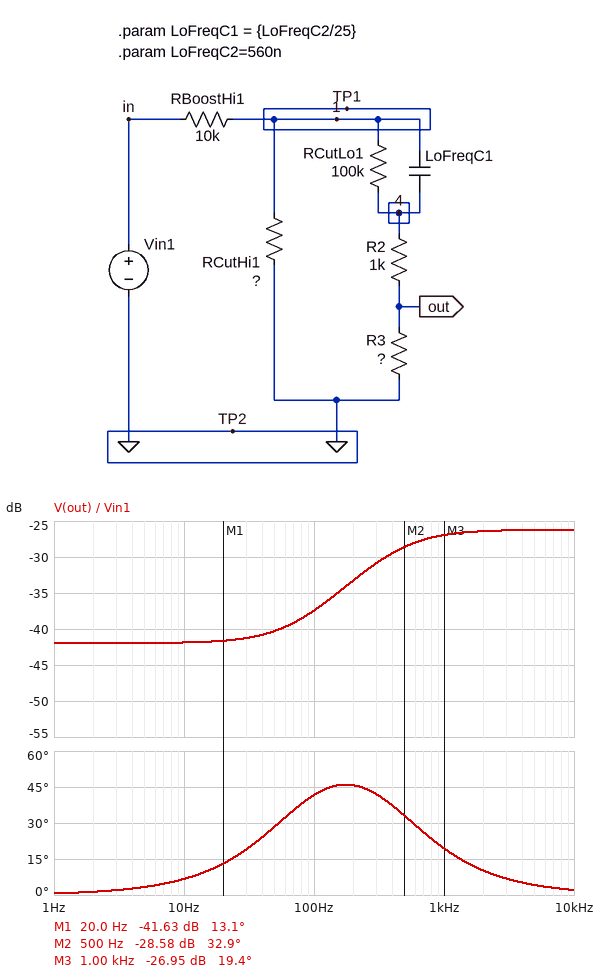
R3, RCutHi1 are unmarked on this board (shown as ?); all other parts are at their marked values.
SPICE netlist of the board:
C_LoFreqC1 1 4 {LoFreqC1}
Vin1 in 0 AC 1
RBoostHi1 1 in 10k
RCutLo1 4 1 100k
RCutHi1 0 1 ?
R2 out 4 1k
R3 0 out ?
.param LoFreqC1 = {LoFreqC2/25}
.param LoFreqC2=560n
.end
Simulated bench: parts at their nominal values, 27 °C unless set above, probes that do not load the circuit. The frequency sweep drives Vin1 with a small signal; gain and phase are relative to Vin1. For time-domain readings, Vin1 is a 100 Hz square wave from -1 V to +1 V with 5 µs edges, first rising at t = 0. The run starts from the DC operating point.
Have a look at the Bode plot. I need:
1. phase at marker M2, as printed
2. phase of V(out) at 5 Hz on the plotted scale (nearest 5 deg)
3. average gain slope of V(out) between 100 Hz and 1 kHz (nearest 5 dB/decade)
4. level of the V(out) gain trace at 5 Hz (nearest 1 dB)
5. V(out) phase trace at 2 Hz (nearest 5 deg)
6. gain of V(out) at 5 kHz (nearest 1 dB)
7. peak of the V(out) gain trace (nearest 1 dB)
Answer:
32.9 deg
5 deg
10 dB/decade
-42 dB
0 deg
-26 dB
-26 dB
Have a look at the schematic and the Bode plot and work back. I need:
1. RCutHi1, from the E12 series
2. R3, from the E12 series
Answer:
560 Ω
18 kΩ
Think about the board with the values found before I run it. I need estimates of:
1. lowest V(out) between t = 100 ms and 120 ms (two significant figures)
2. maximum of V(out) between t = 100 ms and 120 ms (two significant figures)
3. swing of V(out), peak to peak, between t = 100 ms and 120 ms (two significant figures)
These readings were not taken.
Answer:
-89 mV
89 mV
180 mV
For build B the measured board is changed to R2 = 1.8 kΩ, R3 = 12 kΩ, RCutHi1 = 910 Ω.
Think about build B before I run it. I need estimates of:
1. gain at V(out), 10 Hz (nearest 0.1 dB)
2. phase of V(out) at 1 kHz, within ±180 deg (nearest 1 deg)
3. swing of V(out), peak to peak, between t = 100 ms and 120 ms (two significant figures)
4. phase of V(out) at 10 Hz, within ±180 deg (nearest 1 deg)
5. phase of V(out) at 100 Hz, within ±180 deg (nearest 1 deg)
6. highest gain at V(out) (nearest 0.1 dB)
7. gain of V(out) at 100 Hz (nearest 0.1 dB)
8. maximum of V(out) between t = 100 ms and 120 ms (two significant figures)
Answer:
-41.1 dB
25 deg
250 mV
7 deg
44 deg
-23.3 dB
-36.6 dB
130 mV
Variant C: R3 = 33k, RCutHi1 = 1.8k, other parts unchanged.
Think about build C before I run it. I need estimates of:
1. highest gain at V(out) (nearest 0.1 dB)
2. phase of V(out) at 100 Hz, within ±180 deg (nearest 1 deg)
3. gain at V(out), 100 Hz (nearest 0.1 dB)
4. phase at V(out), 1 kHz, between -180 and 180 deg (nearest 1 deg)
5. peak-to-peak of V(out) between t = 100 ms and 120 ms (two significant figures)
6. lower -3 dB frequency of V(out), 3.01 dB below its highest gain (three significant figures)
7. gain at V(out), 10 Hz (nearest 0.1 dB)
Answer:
-17.0 dB
34 deg
-24.4 dB
11 deg
490 mV
252 Hz
-28.5 dB
